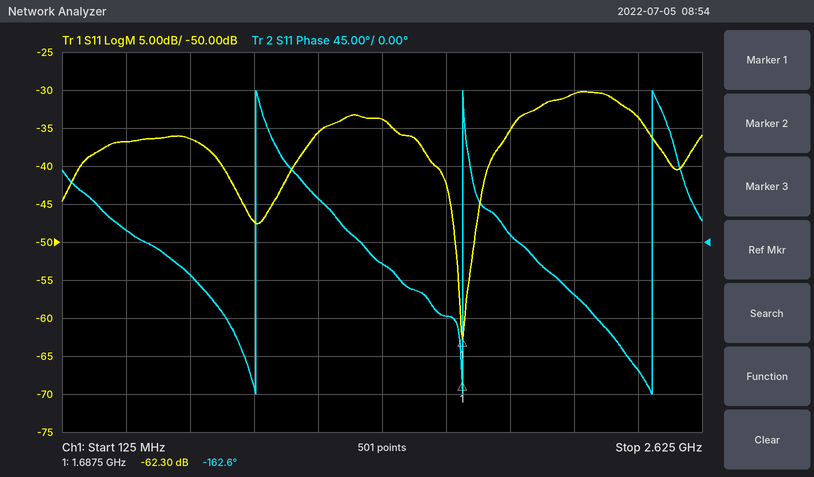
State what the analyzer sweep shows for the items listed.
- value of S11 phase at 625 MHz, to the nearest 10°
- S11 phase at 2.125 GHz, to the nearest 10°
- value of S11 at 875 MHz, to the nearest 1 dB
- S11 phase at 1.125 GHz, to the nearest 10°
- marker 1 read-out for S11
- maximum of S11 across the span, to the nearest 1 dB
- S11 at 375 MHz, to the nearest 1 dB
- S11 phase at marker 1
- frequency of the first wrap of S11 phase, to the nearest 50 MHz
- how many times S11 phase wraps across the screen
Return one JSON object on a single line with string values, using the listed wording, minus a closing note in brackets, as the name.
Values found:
{"value of S11 phase at 625 MHz, to the nearest 10°": "-40°", "S11 phase at 2.125 GHz, to the nearest 10°": "-60°", "value of S11 at 875 MHz, to the nearest 1 dB": "-47 dB", "S11 phase at 1.125 GHz, to the nearest 10°": "50°", "marker 1 read-out for S11": "-62.30 dB", "maximum of S11 across the span, to the nearest 1 dB": "-30 dB", "S11 at 375 MHz, to the nearest 1 dB": "-37 dB", "S11 phase at marker 1": "-162.6°", "frequency of the first wrap of S11 phase, to the nearest 50 MHz": "900 MHz", "how many times S11 phase wraps across the screen": "3"}
